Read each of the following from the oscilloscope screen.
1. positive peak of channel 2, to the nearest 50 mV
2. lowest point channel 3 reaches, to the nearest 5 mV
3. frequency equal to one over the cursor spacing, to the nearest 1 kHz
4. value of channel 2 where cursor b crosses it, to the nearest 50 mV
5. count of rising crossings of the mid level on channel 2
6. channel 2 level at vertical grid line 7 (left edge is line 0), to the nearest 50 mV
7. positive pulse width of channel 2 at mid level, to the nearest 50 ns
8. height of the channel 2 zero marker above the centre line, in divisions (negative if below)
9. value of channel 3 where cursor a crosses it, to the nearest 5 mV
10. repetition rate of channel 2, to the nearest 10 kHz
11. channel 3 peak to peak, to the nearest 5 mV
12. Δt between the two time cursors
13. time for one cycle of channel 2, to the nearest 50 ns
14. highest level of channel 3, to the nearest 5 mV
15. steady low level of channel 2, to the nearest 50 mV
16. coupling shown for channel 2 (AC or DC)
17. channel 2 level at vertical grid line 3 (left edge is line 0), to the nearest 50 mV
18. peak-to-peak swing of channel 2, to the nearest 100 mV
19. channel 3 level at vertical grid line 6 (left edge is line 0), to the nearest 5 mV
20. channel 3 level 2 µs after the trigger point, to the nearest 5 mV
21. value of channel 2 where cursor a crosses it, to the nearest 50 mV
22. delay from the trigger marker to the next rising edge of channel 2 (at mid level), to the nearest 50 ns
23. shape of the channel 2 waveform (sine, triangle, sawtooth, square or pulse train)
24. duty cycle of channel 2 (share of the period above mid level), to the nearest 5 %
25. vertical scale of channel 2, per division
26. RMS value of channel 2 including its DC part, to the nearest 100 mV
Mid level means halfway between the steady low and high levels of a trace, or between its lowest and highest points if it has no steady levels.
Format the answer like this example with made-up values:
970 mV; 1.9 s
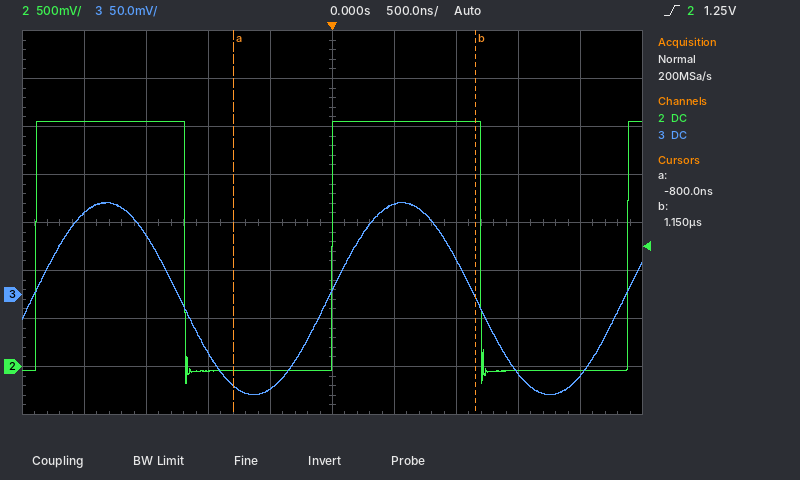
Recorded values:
2.55 V; -105 mV; 513 kHz; 2.55 V; 3; 2.55 V; 1.20 µs; -3.0 div; -95 mV; 420 kHz; 200 mV; 1.95 µs; 2.40 µs; 95 mV; -50 mV; DC; -50 mV; 2.70 V; 95 mV; -85 mV; -50 mV; 2.40 µs; square; 50 %; 500 mV; 1.8 V
